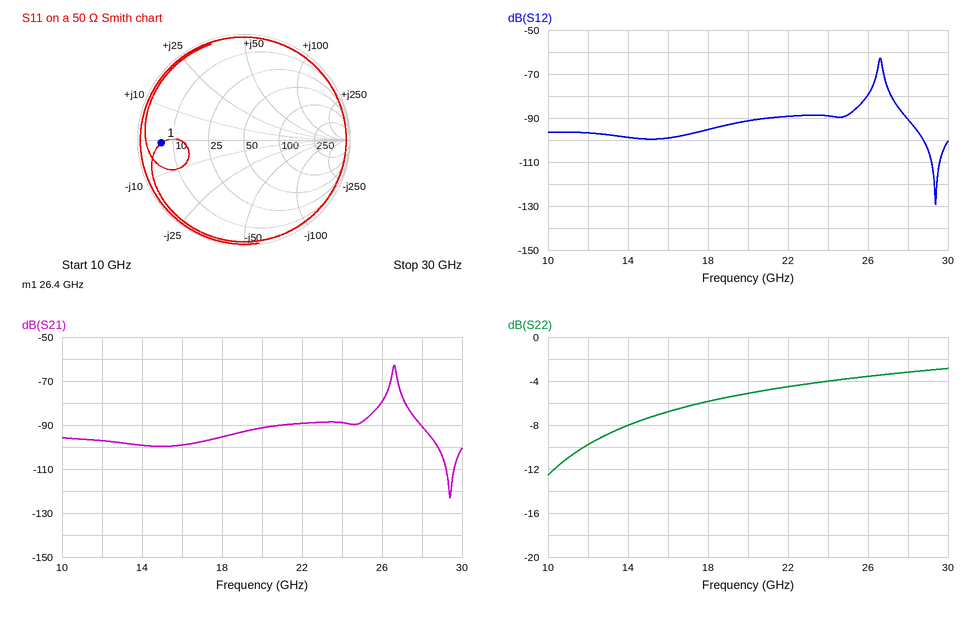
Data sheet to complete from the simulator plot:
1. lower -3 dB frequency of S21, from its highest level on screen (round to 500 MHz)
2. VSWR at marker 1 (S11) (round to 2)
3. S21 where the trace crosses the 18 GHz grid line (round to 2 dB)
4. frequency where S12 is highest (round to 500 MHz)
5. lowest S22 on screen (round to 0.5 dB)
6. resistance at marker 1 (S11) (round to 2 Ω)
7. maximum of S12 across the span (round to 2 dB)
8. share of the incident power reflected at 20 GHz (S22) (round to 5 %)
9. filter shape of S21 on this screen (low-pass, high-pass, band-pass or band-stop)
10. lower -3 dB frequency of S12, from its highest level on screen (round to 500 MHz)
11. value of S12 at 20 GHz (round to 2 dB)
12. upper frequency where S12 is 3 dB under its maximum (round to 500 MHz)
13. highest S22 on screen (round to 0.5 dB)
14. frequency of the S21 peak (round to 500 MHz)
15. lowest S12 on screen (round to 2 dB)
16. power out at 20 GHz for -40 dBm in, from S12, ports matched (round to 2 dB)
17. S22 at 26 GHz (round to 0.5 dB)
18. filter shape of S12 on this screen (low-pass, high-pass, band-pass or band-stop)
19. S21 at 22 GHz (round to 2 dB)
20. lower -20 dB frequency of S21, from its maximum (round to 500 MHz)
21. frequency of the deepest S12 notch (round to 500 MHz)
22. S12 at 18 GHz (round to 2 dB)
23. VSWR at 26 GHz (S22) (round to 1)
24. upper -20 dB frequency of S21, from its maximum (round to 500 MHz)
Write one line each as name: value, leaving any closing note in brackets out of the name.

lower -3 dB frequency of S21, from its highest level on screen: 26.5 GHz
VSWR at marker 1 (S11): 8
S21 where the trace crosses the 18 GHz grid line: -96 dB
frequency where S12 is highest: 26.5 GHz
lowest S22 on screen: -12.5 dB
resistance at marker 1 (S11): 6 Ω
maximum of S12 across the span: -62 dB
share of the incident power reflected at 20 GHz (S22): 30 %
filter shape of S21 on this screen: band-pass
lower -3 dB frequency of S12, from its highest level on screen: 26.5 GHz
value of S12 at 20 GHz: -92 dB
upper frequency where S12 is 3 dB under its maximum: 26.5 GHz
highest S22 on screen: -3.0 dB
frequency of the S21 peak: 26.5 GHz
lowest S12 on screen: -130 dB
power out at 20 GHz for -40 dBm in, from S12, ports matched: -132 dBm
S22 at 26 GHz: -3.5 dB
filter shape of S12 on this screen: band-pass
S21 at 22 GHz: -90 dB
lower -20 dB frequency of S21, from its maximum: 25.5 GHz
frequency of the deepest S12 notch: 29.5 GHz
S12 at 18 GHz: -96 dB
VSWR at 26 GHz (S22): 5
upper -20 dB frequency of S21, from its maximum: 27.5 GHz
